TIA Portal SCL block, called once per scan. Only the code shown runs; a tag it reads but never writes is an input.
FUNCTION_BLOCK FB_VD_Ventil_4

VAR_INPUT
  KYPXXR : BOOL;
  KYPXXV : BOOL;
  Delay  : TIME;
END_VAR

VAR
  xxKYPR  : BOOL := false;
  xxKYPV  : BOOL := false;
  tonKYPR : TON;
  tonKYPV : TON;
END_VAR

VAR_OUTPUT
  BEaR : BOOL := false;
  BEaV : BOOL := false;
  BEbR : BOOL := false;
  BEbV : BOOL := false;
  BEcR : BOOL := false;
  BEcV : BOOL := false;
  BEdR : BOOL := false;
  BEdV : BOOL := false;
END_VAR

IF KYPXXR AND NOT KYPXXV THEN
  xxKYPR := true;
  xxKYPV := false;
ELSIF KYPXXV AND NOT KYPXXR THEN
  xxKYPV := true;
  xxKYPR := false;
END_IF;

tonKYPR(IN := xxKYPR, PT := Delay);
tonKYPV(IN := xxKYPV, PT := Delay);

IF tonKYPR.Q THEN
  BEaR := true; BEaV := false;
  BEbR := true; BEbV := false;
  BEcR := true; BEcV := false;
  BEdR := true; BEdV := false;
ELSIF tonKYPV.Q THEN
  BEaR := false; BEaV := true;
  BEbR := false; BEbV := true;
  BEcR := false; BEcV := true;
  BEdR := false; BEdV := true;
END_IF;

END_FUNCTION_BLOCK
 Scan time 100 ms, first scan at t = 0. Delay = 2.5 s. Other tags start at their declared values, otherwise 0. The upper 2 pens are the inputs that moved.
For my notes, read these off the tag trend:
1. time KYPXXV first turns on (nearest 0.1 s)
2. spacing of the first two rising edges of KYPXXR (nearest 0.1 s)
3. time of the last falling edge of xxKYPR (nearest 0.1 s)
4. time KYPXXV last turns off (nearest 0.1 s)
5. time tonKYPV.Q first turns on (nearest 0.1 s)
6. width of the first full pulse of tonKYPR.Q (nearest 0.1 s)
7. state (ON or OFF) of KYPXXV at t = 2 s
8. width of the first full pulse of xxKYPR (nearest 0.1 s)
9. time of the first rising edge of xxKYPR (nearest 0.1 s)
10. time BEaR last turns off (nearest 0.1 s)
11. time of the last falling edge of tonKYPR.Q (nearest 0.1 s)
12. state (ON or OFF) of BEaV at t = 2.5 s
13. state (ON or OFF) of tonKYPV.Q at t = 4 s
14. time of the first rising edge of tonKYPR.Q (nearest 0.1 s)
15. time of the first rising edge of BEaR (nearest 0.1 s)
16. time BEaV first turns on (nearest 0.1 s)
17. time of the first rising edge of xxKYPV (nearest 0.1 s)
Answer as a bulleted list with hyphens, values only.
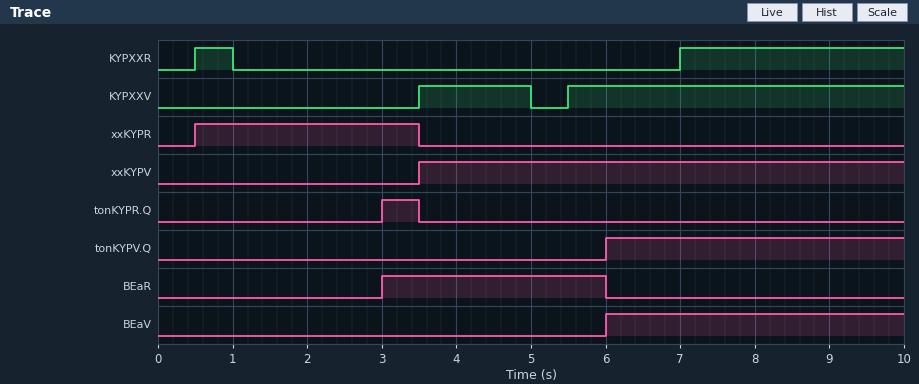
- 3.5 s
- 6.5 s
- 3.5 s
- 5.0 s
- 6.0 s
- 0.5 s
- OFF
- 3.0 s
- 0.5 s
- 6.0 s
- 3.5 s
- OFF
- OFF
- 3.0 s
- 3.0 s
- 6.0 s
- 3.5 s
